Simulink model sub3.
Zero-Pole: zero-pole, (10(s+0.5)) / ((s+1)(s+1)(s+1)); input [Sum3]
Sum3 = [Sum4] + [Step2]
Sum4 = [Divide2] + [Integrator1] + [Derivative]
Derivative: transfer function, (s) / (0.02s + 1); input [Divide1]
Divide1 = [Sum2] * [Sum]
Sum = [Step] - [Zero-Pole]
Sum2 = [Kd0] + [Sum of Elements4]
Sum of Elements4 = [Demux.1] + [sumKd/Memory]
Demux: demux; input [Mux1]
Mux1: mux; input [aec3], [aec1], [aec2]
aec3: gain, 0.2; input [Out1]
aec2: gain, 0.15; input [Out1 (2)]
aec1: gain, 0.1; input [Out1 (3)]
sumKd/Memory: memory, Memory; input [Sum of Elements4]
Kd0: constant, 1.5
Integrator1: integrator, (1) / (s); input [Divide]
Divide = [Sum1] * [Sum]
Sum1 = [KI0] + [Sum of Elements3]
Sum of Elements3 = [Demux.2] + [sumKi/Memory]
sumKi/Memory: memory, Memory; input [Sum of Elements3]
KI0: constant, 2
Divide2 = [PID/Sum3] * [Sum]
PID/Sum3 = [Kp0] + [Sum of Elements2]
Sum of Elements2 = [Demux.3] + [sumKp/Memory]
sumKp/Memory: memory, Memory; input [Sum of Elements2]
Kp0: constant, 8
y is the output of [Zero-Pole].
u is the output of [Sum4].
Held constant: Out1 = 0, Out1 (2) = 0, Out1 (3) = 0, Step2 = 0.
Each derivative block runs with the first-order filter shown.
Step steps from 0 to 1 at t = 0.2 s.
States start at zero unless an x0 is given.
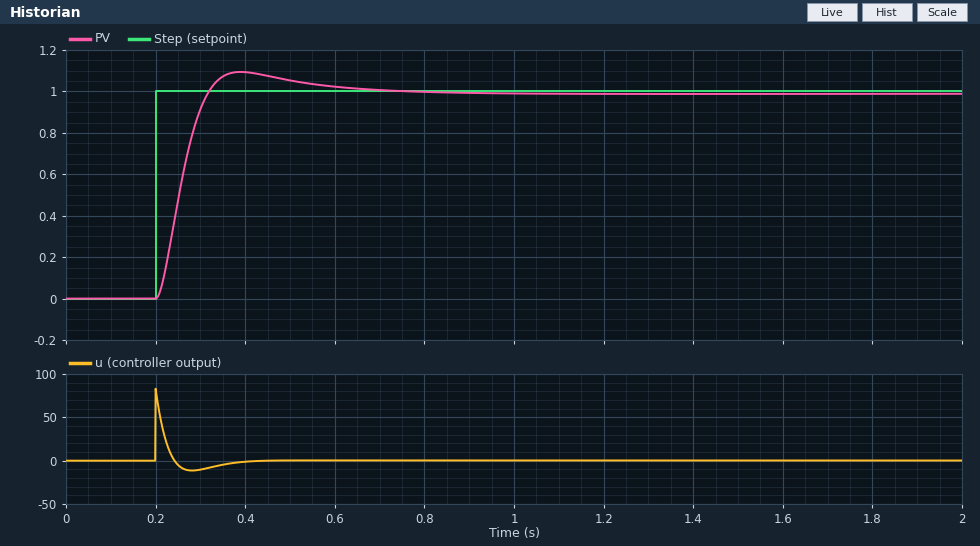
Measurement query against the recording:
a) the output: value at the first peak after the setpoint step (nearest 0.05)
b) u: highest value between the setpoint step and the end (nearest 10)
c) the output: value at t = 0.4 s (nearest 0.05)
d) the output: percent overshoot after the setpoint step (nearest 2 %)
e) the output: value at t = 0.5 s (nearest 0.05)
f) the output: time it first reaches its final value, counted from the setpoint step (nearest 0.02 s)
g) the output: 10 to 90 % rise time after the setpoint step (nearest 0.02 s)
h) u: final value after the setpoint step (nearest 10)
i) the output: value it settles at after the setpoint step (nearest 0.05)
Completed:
1.10
80
1.10
10 %
1.05
0.12 s
0.08 s
0
1.00
